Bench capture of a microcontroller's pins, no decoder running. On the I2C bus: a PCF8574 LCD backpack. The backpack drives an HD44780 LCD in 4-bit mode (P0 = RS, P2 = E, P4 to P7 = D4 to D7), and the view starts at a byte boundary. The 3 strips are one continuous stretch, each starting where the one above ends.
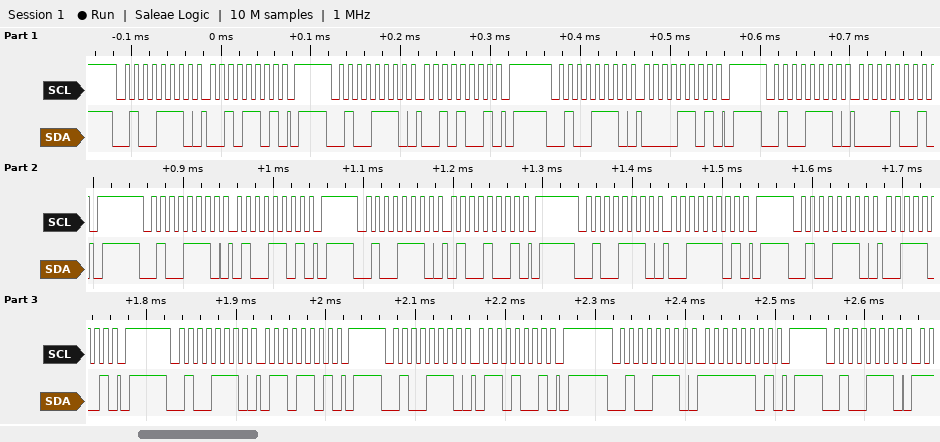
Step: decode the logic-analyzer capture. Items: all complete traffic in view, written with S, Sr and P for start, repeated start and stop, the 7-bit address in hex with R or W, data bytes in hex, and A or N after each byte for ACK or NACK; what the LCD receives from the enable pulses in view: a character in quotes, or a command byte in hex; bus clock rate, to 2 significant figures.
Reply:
S 27W A 2D A P S 27W A 29 A P S 27W A 0D A P S 27W A 09 A P S 27W A 4D A P S 27W A 49 A P S 27W A 3D A P S 27W A 39 A P S 27W A 6D A P S 27W A 69 A P S 27W A FD A P S 27W A
' ' 'C'
100 kHz
